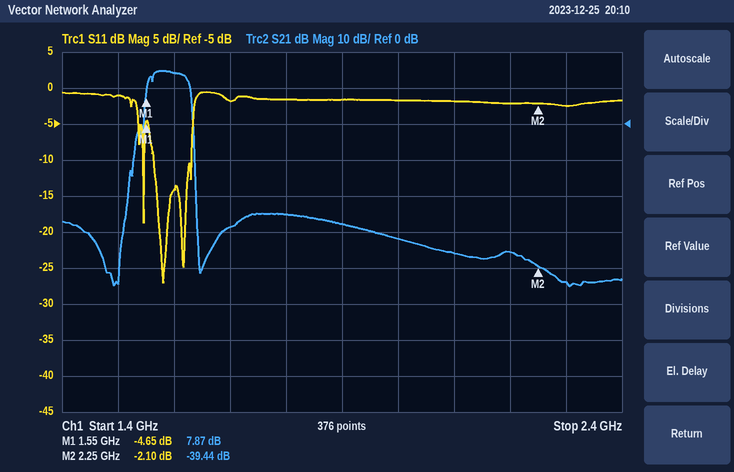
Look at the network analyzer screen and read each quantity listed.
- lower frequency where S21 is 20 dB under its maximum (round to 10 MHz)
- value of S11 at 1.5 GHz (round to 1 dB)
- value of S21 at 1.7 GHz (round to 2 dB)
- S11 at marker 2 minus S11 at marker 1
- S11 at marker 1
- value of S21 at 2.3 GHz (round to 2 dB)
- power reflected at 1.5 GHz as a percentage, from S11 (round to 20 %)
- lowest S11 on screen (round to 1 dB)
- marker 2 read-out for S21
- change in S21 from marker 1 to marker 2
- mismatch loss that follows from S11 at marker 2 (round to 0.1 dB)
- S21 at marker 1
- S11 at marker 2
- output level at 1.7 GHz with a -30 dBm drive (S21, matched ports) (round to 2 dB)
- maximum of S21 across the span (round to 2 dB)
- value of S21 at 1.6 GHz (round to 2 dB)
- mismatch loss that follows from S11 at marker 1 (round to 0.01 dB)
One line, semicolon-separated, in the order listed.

1.53 GHz; -1 dB; -28 dB; 2.55 dB; -4.65 dB; -44 dB; 80 %; -27 dB; -39.44 dB; -47.31 dB; 4.2 dB; 7.87 dB; -2.10 dB; -58 dBm; 14 dB; 14 dB; 1.82 dB
